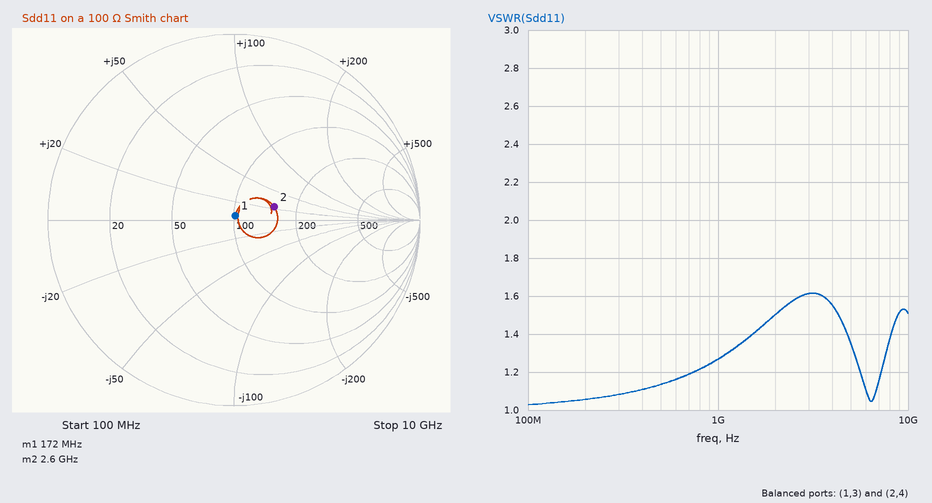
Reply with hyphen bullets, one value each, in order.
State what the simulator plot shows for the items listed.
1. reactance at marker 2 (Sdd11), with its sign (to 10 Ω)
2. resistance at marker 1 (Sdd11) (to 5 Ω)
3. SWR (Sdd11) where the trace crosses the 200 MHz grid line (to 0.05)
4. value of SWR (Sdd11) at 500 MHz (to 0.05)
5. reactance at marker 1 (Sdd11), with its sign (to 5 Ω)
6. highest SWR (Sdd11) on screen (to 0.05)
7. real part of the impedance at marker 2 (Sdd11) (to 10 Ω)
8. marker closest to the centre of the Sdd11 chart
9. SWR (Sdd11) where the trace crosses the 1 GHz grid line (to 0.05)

- +20 Ω
- 100 Ω
- 1.05
- 1.15
- +5 Ω
- 1.60
- 150 Ω
- marker 1
- 1.25
